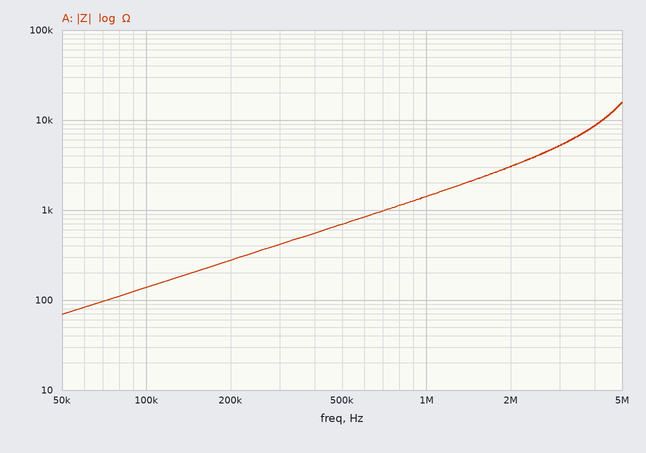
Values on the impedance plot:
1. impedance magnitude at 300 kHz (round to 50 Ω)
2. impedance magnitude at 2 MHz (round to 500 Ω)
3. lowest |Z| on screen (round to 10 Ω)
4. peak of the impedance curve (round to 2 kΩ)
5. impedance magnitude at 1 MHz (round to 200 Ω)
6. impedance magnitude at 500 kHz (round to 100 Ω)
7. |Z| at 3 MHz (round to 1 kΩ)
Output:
400 Ω
3.0 kΩ
70 Ω
16 kΩ
1.4 kΩ
700 Ω
5 kΩ
